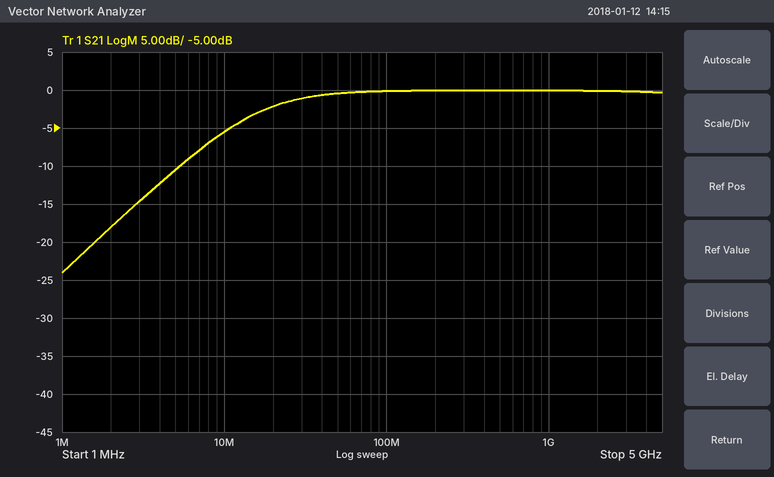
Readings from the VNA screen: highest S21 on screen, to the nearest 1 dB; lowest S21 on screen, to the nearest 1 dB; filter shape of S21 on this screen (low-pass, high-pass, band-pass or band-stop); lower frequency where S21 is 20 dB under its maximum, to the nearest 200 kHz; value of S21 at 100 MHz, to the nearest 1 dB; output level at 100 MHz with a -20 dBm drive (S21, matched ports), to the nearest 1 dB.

0 dB
-24 dB
high-pass
1.6 MHz
0 dB
-20 dBm
